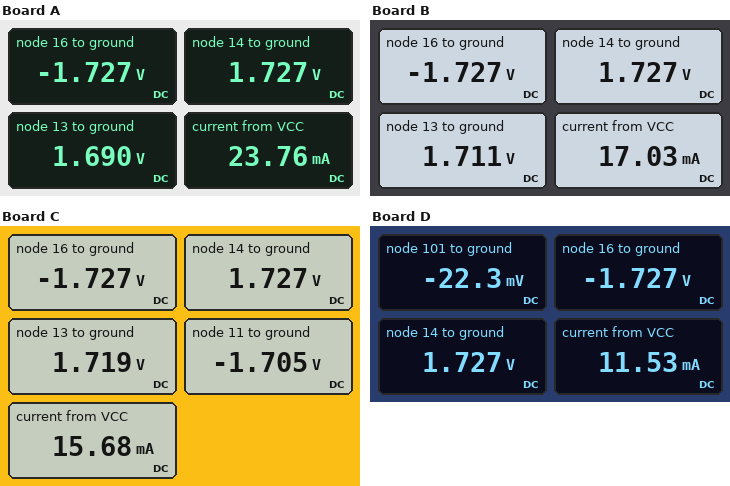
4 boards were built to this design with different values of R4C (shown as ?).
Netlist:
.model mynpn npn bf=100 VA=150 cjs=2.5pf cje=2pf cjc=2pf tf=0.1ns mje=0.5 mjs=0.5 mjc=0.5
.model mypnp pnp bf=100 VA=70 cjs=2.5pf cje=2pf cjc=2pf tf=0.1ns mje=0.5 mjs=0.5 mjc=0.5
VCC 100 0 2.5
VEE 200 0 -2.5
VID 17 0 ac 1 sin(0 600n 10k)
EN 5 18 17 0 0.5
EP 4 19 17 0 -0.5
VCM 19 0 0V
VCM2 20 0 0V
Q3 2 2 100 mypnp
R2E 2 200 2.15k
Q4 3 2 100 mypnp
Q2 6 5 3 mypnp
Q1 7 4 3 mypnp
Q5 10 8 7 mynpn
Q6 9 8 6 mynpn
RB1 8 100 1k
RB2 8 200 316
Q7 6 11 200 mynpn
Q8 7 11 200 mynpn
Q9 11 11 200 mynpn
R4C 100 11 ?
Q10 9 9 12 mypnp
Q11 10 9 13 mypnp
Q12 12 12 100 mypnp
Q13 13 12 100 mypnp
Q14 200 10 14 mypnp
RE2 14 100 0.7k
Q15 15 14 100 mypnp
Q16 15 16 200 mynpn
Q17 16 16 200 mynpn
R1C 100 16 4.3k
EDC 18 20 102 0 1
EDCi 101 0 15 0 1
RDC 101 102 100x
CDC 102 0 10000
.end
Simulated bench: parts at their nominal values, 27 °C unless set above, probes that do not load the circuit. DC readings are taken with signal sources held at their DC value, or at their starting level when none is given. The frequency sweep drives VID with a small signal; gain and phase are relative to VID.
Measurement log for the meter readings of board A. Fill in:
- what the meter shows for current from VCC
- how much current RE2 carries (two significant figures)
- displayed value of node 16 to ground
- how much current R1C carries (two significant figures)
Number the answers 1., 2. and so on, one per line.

1. 23.76 mA
2. 1.1 mA
3. -1.727 V
4. 980 µA
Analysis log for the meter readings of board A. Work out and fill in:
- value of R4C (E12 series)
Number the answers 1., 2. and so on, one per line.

1. 820 Ω
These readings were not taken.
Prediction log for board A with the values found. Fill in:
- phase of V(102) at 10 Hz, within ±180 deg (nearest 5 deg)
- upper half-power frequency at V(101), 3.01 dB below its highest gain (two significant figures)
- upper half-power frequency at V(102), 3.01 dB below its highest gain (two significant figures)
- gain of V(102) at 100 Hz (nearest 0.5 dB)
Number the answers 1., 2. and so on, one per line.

1. 95 deg
2. 89 kHz
3. 580 mHz
4. -44.5 dB
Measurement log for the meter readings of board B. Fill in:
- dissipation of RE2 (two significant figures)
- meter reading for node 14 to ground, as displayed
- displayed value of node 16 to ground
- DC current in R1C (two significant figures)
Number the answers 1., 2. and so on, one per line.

1. 850 µW
2. 1.727 V
3. -1.727 V
4. 980 µA
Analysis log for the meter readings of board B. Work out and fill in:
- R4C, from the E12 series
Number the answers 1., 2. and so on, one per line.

1. 1.5 kΩ
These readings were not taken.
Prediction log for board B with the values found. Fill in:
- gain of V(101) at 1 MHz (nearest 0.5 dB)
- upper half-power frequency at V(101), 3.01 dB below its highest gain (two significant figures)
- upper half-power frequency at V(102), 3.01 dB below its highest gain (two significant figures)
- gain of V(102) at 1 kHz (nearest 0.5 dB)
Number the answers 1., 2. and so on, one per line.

1. 108.5 dB
2. 86 kHz
3. 610 mHz
4. -64.5 dB
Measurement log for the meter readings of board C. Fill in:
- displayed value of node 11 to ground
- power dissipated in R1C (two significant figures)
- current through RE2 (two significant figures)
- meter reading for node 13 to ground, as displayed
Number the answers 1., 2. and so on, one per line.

1. -1.705 V
2. 4.2 mW
3. 1.1 mA
4. 1.719 V
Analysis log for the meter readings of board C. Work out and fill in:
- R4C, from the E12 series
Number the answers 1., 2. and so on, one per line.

1. 1.8 kΩ
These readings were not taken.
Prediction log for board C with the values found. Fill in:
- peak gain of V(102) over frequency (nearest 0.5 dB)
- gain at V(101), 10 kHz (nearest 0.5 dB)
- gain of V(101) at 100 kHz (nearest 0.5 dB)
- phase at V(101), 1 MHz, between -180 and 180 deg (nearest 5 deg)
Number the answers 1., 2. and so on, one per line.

1. 0 dB
2. 131.5 dB
3. 128.0 dB
4. 60 deg
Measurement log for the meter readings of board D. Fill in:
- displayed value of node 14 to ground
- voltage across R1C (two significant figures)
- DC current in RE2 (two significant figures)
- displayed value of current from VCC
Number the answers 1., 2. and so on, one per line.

1. 1.727 V
2. 4.2 V
3. 1.1 mA
4. 11.53 mA
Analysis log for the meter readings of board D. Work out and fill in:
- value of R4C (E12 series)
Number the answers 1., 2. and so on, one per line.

1. 5.6 kΩ
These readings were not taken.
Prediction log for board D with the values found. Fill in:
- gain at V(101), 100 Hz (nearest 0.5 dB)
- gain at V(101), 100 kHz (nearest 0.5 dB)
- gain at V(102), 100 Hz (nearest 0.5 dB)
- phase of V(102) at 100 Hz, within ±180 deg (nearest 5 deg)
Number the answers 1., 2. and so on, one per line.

1. 124.0 dB
2. 120.5 dB
3. -52.0 dB
4. 90 deg
